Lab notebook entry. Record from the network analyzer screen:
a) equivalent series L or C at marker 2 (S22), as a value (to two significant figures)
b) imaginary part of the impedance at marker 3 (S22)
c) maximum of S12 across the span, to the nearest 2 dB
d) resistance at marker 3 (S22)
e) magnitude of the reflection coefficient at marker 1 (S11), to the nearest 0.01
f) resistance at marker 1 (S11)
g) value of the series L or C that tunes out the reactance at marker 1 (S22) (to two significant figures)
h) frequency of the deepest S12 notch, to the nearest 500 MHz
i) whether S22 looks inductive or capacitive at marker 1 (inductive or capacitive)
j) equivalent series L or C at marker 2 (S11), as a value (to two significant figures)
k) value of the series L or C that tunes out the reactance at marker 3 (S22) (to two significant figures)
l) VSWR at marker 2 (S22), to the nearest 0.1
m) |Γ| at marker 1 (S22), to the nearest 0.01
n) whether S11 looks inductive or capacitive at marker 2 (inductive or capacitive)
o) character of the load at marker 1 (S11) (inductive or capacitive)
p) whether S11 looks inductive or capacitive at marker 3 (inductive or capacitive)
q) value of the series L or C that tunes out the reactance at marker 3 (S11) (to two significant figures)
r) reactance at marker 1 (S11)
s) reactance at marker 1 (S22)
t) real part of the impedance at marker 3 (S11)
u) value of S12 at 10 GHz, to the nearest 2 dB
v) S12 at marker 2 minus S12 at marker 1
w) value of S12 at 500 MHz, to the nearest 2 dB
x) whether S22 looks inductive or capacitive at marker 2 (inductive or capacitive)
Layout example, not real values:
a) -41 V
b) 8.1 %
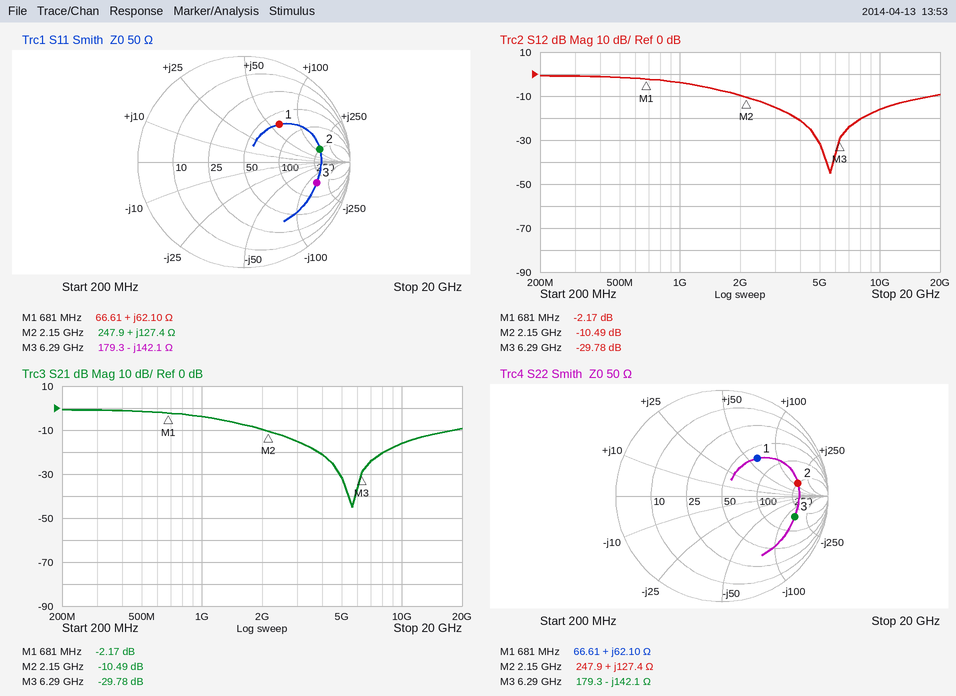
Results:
a) 9.4 nH
b) -142.1 Ω
c) 0 dB
d) 179.3 Ω
e) 0.49
f) 66.61 Ω
g) 3.8 pF
h) 5.5 GHz
i) inductive
j) 9.4 nH
k) 3.6 nH
l) 6.3
m) 0.49
n) inductive
o) inductive
p) capacitive
q) 3.6 nH
r) +62.10 Ω
s) +62.10 Ω
t) 179.3 Ω
u) -16 dB
v) -8.32 dB
w) -2 dB
x) inductive
